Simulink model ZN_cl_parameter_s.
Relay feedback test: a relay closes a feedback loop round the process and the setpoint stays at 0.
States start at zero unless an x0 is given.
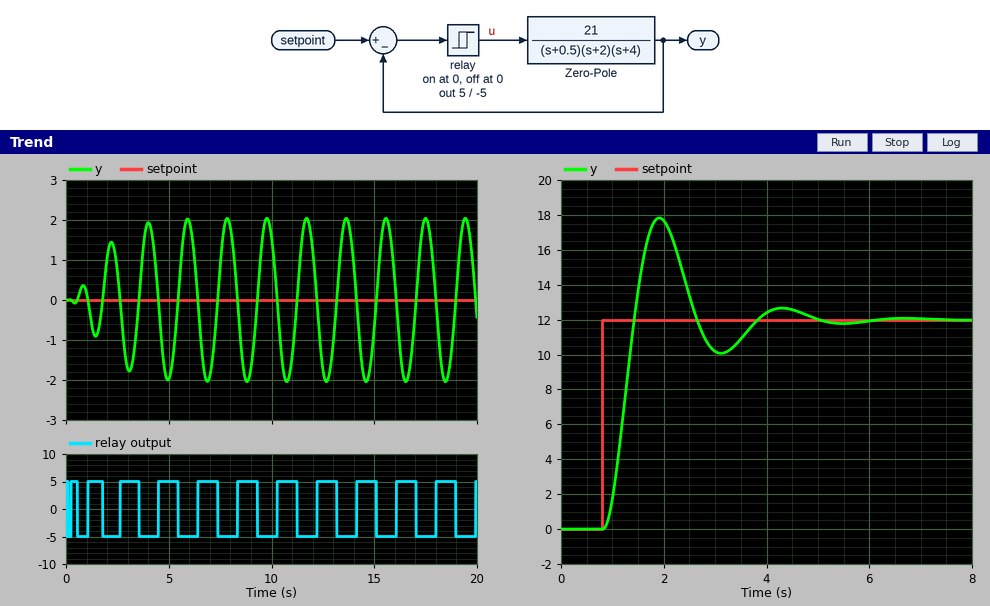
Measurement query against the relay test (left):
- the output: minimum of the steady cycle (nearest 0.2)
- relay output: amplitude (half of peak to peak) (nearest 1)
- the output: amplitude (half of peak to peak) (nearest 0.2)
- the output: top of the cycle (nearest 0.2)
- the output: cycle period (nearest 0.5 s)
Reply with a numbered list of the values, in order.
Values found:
1. -2.0
2. 5
3. 2.0
4. 2.0
5. 2.0 s
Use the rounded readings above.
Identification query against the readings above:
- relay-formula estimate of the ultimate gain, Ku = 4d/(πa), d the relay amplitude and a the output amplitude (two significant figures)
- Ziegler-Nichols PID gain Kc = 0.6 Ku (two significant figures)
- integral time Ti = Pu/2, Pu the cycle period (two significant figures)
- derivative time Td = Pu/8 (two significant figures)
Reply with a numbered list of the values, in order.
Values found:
1. 3.2
2. 1.9
3. 1.0 s
4. 0.25 s
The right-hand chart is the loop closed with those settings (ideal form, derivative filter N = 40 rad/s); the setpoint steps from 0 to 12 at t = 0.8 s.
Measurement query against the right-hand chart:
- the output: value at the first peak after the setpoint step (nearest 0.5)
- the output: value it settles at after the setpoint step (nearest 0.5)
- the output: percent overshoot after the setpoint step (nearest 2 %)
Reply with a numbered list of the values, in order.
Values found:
1. 18.0
2. 12.0
3. 48 %
